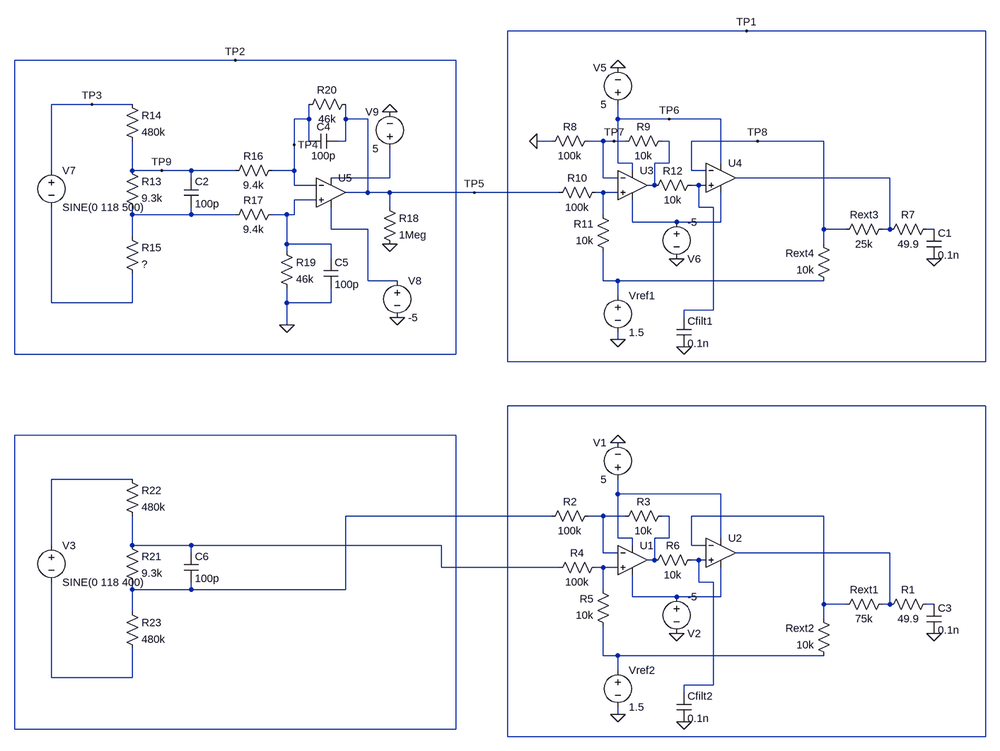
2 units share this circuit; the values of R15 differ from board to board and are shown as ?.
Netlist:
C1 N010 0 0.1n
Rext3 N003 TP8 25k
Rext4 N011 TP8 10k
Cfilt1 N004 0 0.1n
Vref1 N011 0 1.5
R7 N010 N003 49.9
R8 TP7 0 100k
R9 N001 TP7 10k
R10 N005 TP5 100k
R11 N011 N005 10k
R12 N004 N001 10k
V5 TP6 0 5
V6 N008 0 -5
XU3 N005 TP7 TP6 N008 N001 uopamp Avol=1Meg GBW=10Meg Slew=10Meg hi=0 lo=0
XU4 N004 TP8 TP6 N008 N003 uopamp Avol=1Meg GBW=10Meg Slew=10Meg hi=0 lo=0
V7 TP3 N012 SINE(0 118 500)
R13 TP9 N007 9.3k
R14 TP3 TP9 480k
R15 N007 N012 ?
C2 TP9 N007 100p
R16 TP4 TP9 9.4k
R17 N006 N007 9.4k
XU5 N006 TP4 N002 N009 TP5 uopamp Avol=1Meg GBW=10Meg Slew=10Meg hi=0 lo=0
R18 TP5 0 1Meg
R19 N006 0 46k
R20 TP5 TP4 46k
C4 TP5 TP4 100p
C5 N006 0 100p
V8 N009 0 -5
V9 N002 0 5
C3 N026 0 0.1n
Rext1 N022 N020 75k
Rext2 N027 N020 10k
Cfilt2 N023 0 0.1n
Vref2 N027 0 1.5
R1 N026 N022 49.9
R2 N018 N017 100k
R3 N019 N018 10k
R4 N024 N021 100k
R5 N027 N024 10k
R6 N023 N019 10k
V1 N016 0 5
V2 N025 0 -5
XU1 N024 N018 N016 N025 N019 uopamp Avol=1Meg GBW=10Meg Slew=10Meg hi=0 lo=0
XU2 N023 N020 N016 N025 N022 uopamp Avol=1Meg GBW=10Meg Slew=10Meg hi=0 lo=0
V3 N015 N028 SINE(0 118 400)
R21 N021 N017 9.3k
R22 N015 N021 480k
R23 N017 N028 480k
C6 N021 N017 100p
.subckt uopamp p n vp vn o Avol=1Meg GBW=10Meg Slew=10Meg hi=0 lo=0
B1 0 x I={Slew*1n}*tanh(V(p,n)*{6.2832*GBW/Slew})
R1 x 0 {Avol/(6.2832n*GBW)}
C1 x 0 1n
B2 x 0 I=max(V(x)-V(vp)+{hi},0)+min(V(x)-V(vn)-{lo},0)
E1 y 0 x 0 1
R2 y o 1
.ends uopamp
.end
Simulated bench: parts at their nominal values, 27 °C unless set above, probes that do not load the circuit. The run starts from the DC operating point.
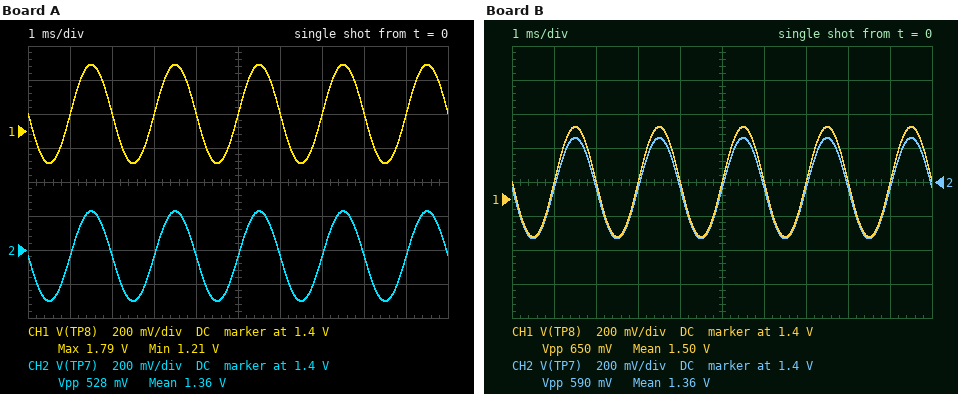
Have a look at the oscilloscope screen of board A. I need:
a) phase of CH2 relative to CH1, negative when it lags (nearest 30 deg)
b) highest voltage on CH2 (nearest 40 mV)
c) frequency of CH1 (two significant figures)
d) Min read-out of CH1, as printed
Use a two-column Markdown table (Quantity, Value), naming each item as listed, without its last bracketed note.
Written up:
| Quantity | Value |
|---|---|
| phase of CH2 relative to CH1, negative when it lags | 0 deg |
| highest voltage on CH2 | 1.64 V |
| frequency of CH1 | 500 Hz |
| Min read-out of CH1, as printed | 1.21 V |
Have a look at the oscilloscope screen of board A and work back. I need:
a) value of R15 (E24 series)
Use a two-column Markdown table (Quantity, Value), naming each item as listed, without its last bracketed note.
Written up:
| Quantity | Value |
|---|---|
| value of R15 | 750 kΩ |
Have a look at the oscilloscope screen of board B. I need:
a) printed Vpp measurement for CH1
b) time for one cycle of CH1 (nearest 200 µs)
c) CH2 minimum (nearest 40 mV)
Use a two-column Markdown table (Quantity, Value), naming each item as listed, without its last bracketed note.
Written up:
| Quantity | Value |
|---|---|
| printed Vpp measurement for CH1 | 650 mV |
| time for one cycle of CH1 | 2.0 ms |
| CH2 minimum | 1.08 V |
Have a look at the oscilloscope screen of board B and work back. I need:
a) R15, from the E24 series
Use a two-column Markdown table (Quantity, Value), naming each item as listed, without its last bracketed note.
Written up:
| Quantity | Value |
|---|---|
| R15, from the E24 series | 620 kΩ |
